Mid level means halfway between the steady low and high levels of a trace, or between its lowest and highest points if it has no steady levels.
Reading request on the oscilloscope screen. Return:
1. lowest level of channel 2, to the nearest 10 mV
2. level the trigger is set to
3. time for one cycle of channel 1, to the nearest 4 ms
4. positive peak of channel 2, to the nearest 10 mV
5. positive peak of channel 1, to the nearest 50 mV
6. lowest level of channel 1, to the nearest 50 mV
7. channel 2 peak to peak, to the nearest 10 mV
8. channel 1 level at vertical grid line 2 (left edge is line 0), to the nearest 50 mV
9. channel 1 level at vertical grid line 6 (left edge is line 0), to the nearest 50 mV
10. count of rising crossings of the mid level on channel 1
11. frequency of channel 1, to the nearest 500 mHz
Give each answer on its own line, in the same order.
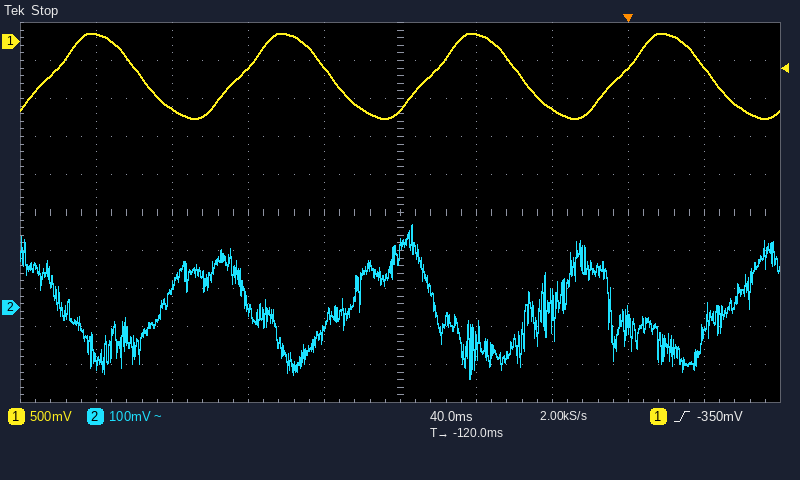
-190 mV
-350 mV
100 ms
220 mV
100 mV
-1.00 V
410 mV
-900 mV
100 mV
4
10.0 Hz
